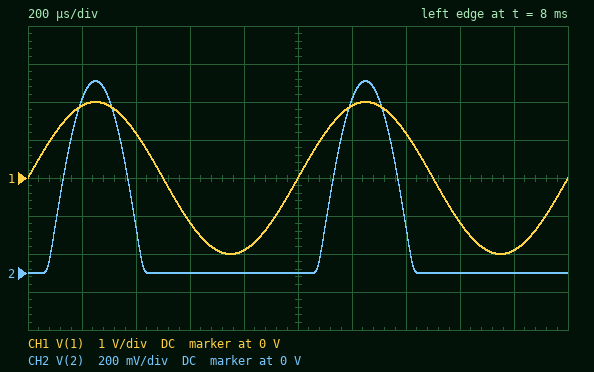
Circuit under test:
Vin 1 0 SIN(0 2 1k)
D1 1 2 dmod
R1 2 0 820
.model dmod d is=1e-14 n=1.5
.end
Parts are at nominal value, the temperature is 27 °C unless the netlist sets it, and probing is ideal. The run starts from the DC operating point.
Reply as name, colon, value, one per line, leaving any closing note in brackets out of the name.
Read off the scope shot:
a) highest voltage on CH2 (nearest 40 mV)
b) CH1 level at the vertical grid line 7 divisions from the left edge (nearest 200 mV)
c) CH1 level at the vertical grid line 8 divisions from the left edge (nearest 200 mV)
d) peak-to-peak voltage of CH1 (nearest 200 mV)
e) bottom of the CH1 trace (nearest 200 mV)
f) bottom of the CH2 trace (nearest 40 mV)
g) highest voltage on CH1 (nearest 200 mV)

highest voltage on CH2: 1.00 V
CH1 level at the vertical grid line 7 divisions from the left edge: 1.2 V
CH1 level at the vertical grid line 8 divisions from the left edge: -1.2 V
peak-to-peak voltage of CH1: 4.0 V
bottom of the CH1 trace: -2.0 V
bottom of the CH2 trace: 0 V
highest voltage on CH1: 2.0 V
